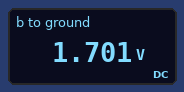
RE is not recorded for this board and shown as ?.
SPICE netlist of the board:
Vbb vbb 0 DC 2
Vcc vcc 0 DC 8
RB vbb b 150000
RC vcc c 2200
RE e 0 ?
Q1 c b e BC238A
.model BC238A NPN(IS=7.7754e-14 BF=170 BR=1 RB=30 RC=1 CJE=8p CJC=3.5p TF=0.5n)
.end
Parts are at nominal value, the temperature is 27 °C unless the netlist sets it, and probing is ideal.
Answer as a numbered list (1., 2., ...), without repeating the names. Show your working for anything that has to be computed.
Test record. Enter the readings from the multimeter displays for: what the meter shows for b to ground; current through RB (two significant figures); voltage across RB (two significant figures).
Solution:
1. 1.701 V
2. (2 V - 1.701 V) / 150 kΩ = 2.0 µA
3. 2 V - 1.701 V = 300 mV
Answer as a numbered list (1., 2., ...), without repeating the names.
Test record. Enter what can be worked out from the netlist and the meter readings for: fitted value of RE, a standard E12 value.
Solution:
1. 3.3 kΩ
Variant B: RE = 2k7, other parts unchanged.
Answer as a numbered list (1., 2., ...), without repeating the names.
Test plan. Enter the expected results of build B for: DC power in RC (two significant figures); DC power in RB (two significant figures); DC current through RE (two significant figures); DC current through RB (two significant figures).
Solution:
1. 340 µW
2. 810 nW
3. 400 µA
4. 2.3 µA
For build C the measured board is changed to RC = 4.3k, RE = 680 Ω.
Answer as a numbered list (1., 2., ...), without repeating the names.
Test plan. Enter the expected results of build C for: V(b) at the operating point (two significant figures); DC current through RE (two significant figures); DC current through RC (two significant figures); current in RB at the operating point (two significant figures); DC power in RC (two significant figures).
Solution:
1. 1.2 V
2. 900 µA
3. 890 µA
4. 5.3 µA
5. 3.4 mW
